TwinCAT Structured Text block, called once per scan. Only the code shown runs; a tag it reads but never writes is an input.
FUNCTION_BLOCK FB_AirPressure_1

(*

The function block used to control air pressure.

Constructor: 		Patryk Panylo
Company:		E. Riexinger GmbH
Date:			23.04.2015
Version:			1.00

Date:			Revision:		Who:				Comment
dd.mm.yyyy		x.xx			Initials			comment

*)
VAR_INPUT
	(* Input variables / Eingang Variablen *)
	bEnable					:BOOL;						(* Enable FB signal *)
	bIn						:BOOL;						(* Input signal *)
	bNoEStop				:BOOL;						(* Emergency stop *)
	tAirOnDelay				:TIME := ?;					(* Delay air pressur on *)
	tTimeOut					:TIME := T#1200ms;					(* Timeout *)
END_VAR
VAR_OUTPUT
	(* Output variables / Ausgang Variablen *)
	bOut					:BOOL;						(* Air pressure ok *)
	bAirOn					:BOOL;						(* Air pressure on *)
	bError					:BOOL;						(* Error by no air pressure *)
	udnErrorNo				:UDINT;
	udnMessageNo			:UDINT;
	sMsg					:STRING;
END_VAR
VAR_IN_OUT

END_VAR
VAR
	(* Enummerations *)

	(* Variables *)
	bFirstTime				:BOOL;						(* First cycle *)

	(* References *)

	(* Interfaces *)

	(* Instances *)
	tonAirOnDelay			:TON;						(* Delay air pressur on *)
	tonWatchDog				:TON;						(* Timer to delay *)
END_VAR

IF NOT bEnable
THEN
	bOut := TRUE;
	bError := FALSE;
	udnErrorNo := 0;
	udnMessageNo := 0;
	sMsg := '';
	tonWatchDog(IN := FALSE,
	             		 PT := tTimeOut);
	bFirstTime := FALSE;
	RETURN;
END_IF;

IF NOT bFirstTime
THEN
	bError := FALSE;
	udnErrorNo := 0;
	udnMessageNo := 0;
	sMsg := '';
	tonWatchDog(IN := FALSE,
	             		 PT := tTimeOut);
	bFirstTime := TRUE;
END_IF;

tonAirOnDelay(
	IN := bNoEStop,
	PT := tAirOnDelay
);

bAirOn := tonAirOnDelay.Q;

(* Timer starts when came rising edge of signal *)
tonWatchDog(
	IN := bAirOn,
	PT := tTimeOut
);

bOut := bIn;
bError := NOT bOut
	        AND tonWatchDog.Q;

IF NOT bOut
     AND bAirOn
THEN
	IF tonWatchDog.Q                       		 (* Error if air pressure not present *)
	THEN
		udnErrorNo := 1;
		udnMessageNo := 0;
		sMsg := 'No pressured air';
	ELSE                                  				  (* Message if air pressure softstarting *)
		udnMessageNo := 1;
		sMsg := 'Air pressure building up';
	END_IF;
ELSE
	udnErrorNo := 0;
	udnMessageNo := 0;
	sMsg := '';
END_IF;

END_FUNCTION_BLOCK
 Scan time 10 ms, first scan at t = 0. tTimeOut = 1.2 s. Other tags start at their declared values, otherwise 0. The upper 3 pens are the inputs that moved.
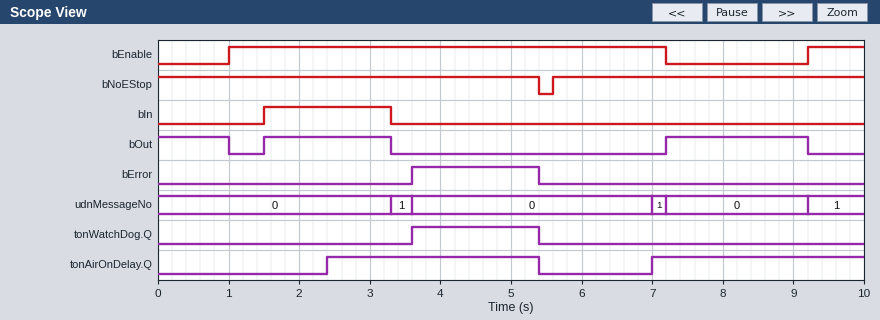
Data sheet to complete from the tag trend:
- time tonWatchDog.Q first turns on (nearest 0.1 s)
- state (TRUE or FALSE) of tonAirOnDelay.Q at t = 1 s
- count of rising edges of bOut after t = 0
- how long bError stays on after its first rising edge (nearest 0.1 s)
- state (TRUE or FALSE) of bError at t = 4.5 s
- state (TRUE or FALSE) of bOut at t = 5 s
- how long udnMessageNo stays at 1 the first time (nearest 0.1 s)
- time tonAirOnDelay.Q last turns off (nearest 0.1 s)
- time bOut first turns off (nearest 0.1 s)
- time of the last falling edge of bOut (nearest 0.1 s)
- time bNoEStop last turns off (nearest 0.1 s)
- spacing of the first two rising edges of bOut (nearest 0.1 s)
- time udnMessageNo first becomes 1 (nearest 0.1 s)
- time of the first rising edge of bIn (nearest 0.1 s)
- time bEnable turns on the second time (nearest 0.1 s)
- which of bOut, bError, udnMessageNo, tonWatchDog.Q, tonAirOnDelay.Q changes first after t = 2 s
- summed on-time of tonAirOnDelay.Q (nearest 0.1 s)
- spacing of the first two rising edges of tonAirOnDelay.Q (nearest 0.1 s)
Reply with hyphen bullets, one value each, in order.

- 3.6 s
- FALSE
- 2
- 1.8 s
- TRUE
- FALSE
- 0.3 s
- 5.4 s
- 1.0 s
- 9.2 s
- 5.4 s
- 5.7 s
- 3.3 s
- 1.5 s
- 9.2 s
- tonAirOnDelay.Q
- 6.0 s
- 4.6 s
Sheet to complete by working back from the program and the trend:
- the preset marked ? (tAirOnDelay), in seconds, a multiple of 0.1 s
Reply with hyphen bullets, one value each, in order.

- 1.4 s
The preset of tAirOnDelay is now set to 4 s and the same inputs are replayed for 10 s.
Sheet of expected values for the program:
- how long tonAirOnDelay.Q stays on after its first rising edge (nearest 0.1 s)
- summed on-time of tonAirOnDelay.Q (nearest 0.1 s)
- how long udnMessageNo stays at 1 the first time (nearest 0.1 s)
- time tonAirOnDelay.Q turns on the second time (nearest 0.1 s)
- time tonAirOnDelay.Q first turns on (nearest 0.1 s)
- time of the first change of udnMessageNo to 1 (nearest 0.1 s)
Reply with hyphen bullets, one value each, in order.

- 0.4 s
- 0.8 s
- 0.4 s
- 9.6 s
- 5.0 s
- 5.0 s
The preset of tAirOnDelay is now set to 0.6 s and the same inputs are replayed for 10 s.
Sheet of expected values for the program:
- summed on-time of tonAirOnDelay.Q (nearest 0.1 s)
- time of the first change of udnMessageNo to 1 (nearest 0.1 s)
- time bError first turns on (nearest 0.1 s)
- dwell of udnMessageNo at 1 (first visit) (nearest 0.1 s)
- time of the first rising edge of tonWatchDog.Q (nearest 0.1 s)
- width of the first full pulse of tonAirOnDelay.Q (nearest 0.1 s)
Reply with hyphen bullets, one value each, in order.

- 7.6 s
- 6.2 s
- 3.3 s
- 1.0 s
- 2.8 s
- 3.8 s
